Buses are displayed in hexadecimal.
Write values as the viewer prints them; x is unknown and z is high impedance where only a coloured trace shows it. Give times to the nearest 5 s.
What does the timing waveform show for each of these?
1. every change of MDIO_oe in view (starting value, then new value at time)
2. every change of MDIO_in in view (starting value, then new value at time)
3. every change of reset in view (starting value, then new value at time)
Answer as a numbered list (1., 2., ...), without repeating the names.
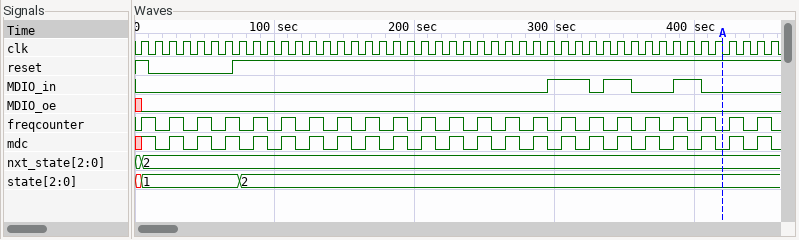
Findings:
1. x, 0 at 5 s
2. 0, 1 at 295 s, 0 at 325 s, 1 at 335 s, 0 at 355 s, 1 at 385 s, 0 at 405 s
3. 1, 0 at 10 s, 1 at 70 s
